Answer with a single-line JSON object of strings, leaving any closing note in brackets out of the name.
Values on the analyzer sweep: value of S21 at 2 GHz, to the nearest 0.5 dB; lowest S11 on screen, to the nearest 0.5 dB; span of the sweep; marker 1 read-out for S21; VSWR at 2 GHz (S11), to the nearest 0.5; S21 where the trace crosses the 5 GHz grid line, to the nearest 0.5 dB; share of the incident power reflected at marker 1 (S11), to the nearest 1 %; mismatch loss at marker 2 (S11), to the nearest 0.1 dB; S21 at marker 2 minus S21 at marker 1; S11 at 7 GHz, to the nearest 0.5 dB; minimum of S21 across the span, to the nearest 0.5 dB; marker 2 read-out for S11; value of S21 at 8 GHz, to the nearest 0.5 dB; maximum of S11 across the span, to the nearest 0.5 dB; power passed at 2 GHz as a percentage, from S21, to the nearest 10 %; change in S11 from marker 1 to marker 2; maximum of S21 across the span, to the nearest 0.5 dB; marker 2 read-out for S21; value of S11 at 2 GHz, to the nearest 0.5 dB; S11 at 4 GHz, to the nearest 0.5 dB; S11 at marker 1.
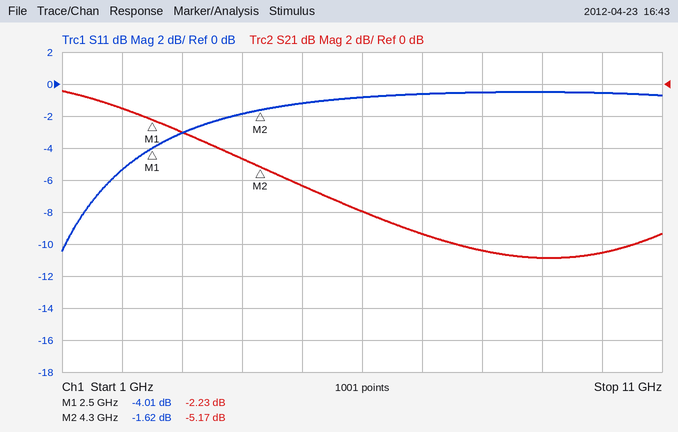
{"value of S21 at 2 GHz, to the nearest 0.5 dB": "-1.5 dB", "lowest S11 on screen, to the nearest 0.5 dB": "-10.5 dB", "span of the sweep": "10 GHz", "marker 1 read-out for S21": "-2.23 dB", "VSWR at 2 GHz (S11), to the nearest 0.5": "3.5", "S21 where the trace crosses the 5 GHz grid line, to the nearest 0.5 dB": "-6.5 dB", "share of the incident power reflected at marker 1 (S11), to the nearest 1 %": "40 %", "mismatch loss at marker 2 (S11), to the nearest 0.1 dB": "5.1 dB", "S21 at marker 2 minus S21 at marker 1": "-2.94 dB", "S11 at 7 GHz, to the nearest 0.5 dB": "-0.5 dB", "minimum of S21 across the span, to the nearest 0.5 dB": "-11.0 dB", "marker 2 read-out for S11": "-1.62 dB", "value of S21 at 8 GHz, to the nearest 0.5 dB": "-10.5 dB", "maximum of S11 across the span, to the nearest 0.5 dB": "-0.5 dB", "power passed at 2 GHz as a percentage, from S21, to the nearest 10 %": "70 %", "change in S11 from marker 1 to marker 2": "2.39 dB", "maximum of S21 across the span, to the nearest 0.5 dB": "-0.5 dB", "marker 2 read-out for S21": "-5.17 dB", "value of S11 at 2 GHz, to the nearest 0.5 dB": "-5.5 dB", "S11 at 4 GHz, to the nearest 0.5 dB": "-2.0 dB", "S11 at marker 1": "-4.01 dB"}
